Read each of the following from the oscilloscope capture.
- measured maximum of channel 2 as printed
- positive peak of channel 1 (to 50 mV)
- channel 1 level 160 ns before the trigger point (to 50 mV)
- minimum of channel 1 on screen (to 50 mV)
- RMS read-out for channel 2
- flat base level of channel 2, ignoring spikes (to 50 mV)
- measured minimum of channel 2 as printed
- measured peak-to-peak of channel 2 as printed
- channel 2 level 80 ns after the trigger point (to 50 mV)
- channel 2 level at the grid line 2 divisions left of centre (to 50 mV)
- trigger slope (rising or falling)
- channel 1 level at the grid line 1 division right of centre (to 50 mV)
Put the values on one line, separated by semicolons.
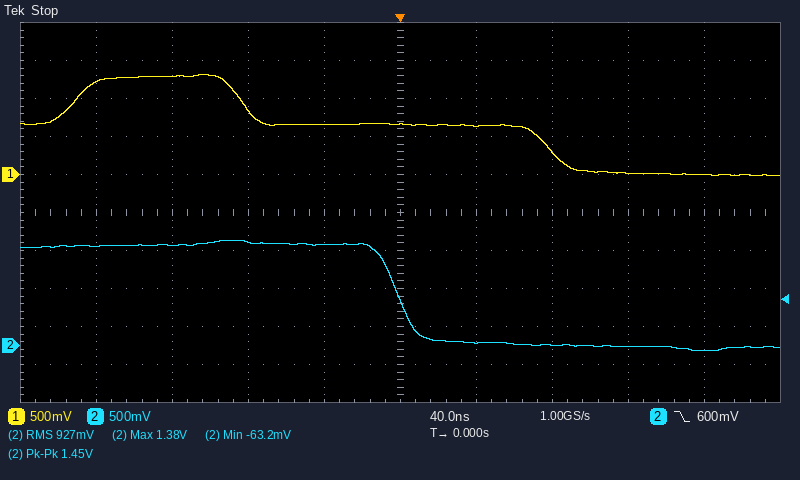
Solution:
1.38 V; 1.30 V; 1.20 V; 0 mV; 927 mV; 0 mV; -63.2 mV; 1.45 V; 0 mV; 1.35 V; falling; 650 mV
